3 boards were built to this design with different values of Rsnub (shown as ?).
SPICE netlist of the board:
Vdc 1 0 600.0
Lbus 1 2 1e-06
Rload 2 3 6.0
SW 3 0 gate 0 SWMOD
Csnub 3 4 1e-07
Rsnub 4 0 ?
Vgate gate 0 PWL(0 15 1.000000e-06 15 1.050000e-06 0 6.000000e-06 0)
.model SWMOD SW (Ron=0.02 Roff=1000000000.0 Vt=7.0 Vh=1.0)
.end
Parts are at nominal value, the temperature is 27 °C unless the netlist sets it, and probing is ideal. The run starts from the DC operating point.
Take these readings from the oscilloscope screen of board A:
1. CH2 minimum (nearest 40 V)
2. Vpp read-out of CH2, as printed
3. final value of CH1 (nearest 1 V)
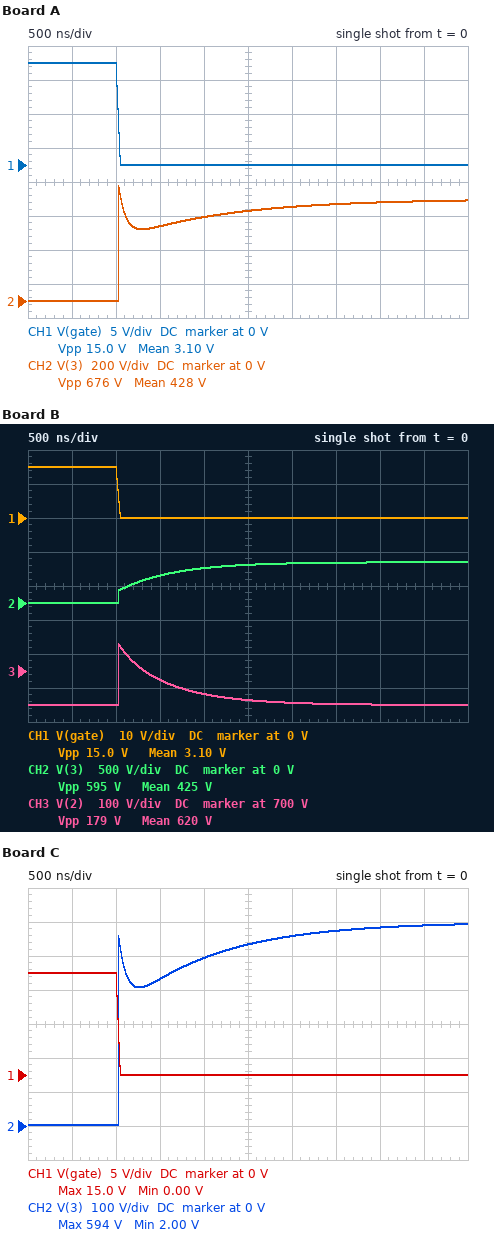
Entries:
0 V
676 V
0 V
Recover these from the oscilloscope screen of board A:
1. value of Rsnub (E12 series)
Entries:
6.8 Ω
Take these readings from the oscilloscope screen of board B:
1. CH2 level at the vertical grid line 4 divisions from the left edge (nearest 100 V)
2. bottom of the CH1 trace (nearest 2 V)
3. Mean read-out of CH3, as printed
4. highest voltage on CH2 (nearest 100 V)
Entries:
500 V
0 V
620 V
600 V
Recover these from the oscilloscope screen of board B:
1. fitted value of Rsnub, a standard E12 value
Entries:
1.8 Ω
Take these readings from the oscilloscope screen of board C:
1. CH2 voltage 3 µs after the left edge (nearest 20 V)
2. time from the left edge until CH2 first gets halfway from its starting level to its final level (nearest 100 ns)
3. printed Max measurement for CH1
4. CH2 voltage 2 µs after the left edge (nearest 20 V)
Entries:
560 V
1.0 µs
15.0 V
500 V
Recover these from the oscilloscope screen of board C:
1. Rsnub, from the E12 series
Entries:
5.6 Ω
